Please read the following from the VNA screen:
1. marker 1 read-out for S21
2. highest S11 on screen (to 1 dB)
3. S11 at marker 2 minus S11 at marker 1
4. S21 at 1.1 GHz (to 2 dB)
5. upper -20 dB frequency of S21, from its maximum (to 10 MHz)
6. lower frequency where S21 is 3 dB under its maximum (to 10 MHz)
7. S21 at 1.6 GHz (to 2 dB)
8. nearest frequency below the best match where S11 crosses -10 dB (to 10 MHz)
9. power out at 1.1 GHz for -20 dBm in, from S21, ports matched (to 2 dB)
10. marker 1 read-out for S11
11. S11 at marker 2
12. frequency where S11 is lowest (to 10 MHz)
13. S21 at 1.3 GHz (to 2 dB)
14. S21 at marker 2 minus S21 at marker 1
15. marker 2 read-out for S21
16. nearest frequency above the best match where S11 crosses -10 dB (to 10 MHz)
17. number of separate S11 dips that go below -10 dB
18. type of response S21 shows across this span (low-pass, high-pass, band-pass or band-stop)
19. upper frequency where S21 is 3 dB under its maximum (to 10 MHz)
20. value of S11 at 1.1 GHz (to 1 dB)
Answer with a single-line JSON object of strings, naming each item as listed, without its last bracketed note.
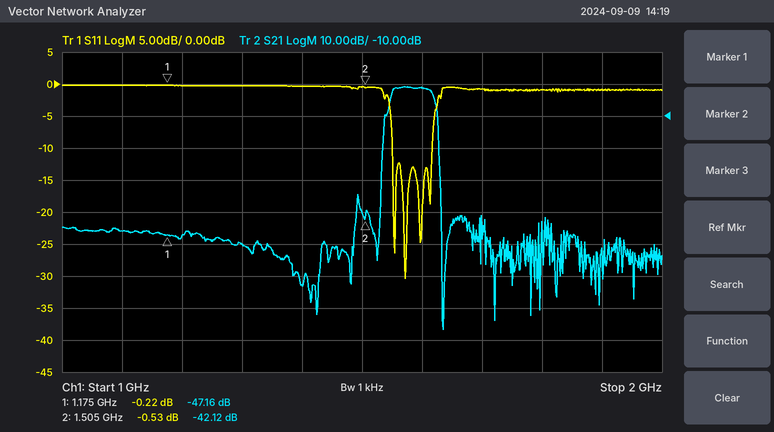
{"marker 1 read-out for S21": "-47.16 dB", "highest S11 on screen": "0 dB", "S11 at marker 2 minus S11 at marker 1": "-0.31 dB", "S21 at 1.1 GHz": "-46 dB", "upper -20 dB frequency of S21, from its maximum": "1.63 GHz", "lower frequency where S21 is 3 dB under its maximum": "1.55 GHz", "S21 at 1.6 GHz": "-2 dB", "nearest frequency below the best match where S11 crosses -10 dB": "1.55 GHz", "power out at 1.1 GHz for -20 dBm in, from S21, ports matched": "-66 dBm", "marker 1 read-out for S11": "-0.22 dB", "S11 at marker 2": "-0.53 dB", "frequency where S11 is lowest": "1.57 GHz", "S21 at 1.3 GHz": "-50 dB", "S21 at marker 2 minus S21 at marker 1": "5.04 dB", "marker 2 read-out for S21": "-42.12 dB", "nearest frequency above the best match where S11 crosses -10 dB": "1.62 GHz", "number of separate S11 dips that go below -10 dB": "4", "type of response S21 shows across this span": "band-pass", "upper frequency where S21 is 3 dB under its maximum": "1.62 GHz", "value of S11 at 1.1 GHz": "0 dB"}
